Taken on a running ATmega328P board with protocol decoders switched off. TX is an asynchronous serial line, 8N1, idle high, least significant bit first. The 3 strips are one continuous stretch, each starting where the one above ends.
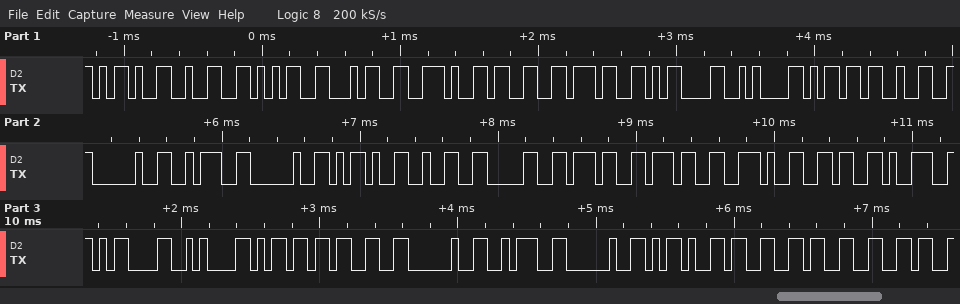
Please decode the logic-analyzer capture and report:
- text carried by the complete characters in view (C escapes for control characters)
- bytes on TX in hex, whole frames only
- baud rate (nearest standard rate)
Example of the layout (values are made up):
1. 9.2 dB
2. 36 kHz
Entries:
1. "-254.37\r\nm2 : -2077.69\r\nm3 : -336"
2. 0x2D 0x32 0x35 0x34 0x2E 0x33 0x37 0x0D 0x0A 0x6D 0x32 0x20 0x3A 0x20 0x2D 0x32 0x30 0x37 0x37 0x2E 0x36 0x39 0x0D 0x0A 0x6D 0x33 0x20 0x3A 0x20 0x2D 0x33 0x33 0x36
3. 19200 baud
